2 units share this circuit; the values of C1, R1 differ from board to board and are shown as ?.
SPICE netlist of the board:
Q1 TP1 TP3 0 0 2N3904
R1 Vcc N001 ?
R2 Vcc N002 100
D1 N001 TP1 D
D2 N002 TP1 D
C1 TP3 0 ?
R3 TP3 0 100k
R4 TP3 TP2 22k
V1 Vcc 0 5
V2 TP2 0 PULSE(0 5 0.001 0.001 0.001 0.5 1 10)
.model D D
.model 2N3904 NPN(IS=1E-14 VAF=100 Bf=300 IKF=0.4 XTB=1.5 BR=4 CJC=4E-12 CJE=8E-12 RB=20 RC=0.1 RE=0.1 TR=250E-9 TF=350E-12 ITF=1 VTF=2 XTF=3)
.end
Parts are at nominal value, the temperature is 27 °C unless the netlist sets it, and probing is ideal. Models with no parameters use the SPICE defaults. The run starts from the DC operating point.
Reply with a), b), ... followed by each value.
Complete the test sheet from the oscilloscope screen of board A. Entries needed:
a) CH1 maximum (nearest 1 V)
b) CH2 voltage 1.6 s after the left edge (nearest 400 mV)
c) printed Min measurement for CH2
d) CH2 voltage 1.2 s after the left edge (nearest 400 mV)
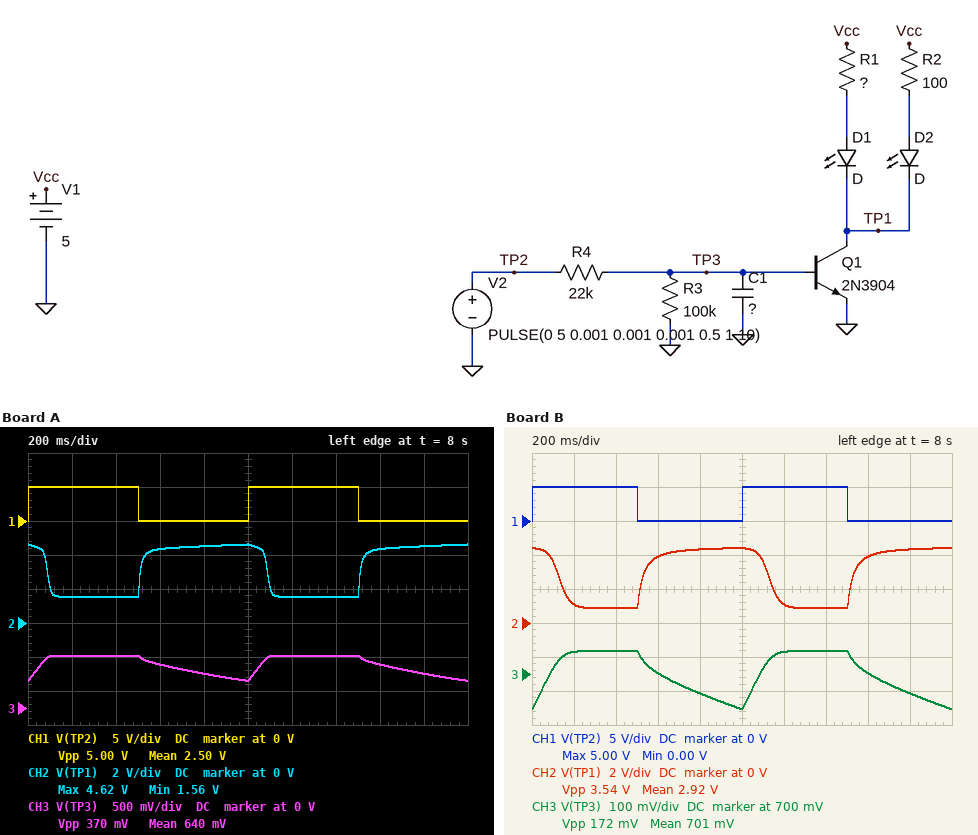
a) 5 V
b) 4.4 V
c) 1.56 V
d) 1.6 V
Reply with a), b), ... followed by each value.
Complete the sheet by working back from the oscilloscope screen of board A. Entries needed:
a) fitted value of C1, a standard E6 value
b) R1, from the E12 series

a) 47 µF
b) 120 Ω
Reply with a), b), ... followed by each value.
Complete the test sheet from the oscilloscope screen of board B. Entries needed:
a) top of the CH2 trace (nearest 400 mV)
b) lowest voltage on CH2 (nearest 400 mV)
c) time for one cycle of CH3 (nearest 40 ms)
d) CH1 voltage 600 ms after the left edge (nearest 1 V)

a) 4.4 V
b) 800 mV
c) 1.00 s
d) 0 V
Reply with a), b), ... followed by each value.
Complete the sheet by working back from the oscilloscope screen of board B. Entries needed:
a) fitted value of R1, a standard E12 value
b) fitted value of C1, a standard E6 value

a) 220 Ω
b) 150 µF
